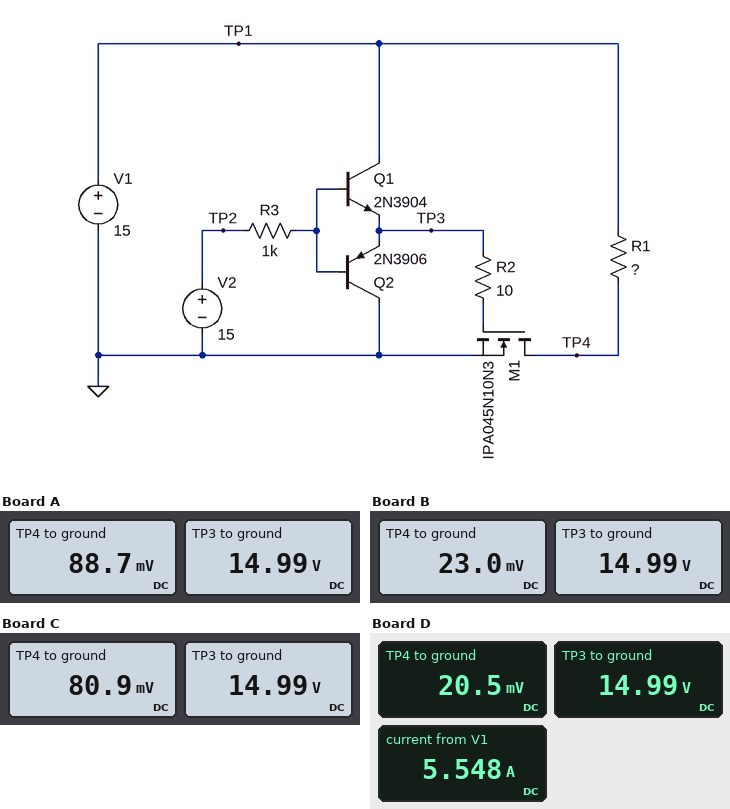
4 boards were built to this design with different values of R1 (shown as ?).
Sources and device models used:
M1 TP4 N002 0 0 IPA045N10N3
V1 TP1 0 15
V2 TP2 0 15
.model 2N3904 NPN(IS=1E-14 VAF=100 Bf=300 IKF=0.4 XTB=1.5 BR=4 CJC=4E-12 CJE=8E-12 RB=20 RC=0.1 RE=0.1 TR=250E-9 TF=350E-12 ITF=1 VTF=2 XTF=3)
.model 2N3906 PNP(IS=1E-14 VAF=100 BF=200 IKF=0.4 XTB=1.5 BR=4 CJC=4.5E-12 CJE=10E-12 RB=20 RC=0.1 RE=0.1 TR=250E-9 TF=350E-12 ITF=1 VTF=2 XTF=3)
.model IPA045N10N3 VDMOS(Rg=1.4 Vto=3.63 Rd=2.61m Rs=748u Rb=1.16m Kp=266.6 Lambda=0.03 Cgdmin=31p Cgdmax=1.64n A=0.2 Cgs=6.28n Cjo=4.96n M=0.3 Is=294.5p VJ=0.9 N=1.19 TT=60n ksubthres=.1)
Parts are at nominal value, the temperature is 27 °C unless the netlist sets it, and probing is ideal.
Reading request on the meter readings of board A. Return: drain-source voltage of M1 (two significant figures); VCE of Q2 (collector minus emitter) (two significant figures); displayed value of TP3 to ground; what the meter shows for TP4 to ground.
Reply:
89 mV
-15 V
14.99 V
88.7 mV
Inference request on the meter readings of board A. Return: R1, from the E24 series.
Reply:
0.62 Ω
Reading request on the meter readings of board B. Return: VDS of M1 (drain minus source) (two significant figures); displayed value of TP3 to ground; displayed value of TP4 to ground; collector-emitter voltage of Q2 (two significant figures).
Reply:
23 mV
14.99 V
23.0 mV
-15 V
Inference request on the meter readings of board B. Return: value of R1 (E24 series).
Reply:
2.4 Ω
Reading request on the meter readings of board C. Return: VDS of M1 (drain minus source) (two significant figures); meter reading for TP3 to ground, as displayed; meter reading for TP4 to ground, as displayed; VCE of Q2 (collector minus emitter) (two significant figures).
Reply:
81 mV
14.99 V
80.9 mV
-15 V
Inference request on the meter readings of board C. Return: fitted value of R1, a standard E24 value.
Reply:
0.68 Ω
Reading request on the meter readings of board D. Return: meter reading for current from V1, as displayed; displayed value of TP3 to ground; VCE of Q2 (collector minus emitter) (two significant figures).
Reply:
5.548 A
14.99 V
-15 V
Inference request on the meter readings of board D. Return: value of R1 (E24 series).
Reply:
2.7 Ω
